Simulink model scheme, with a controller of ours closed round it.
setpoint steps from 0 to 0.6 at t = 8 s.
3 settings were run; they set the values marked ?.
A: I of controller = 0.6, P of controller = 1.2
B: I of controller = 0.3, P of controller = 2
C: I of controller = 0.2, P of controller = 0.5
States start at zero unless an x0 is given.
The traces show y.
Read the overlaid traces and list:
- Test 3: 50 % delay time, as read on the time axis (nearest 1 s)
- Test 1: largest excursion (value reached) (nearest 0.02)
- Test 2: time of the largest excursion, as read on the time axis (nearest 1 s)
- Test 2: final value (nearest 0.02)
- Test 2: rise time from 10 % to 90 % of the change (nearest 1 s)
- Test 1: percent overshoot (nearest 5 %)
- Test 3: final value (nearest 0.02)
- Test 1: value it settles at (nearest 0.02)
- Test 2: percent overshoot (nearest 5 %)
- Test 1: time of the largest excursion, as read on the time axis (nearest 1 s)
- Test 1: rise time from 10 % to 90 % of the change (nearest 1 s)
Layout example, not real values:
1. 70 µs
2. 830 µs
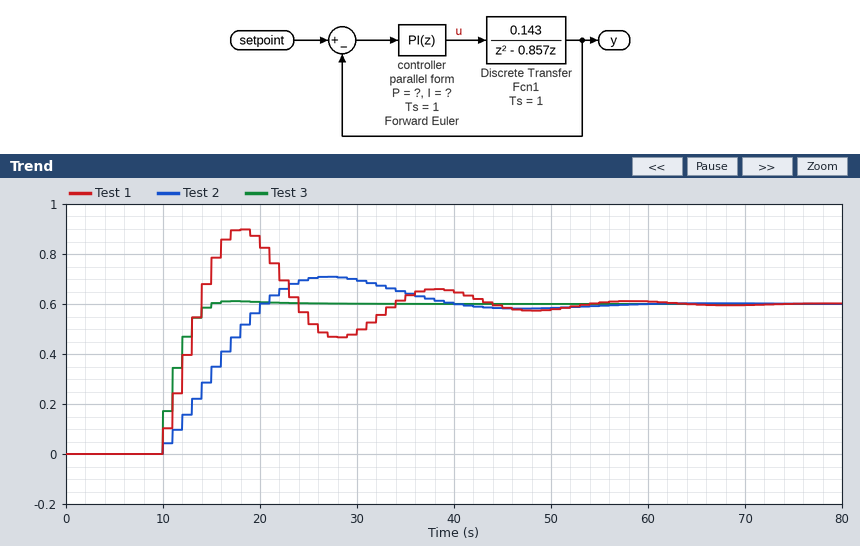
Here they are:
1. 11 s
2. 0.90
3. 27 s
4. 0.60
5. 8 s
6. 50 %
7. 0.60
8. 0.60
9. 20 %
10. 18 s
11. 3 s
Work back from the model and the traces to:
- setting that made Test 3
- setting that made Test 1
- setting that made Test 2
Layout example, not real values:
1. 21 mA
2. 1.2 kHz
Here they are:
1. B
2. A
3. C
